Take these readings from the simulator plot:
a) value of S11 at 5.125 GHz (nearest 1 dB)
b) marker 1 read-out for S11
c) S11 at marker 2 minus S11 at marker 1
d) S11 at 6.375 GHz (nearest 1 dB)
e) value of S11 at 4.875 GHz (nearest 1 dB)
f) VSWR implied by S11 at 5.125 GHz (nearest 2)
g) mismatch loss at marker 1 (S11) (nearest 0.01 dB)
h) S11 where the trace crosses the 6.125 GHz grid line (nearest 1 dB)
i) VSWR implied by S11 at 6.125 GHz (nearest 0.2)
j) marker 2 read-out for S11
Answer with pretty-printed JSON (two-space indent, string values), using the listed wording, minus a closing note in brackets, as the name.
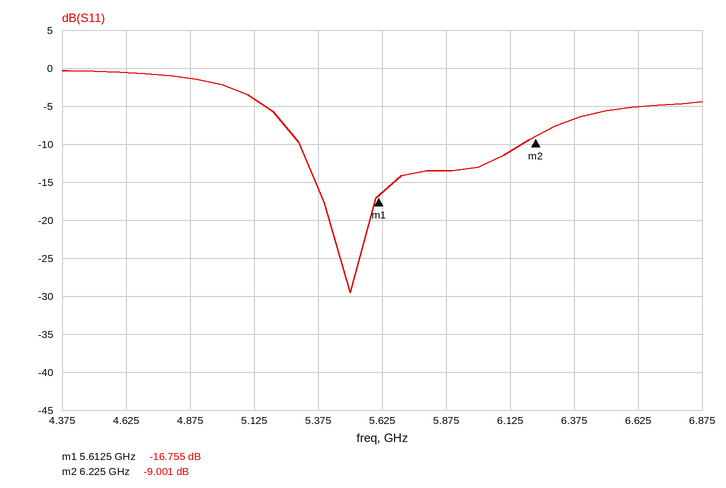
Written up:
{
  "value of S11 at 5.125 GHz": "-4 dB",
  "marker 1 read-out for S11": "-16.755 dB",
  "S11 at marker 2 minus S11 at marker 1": "7.754 dB",
  "S11 at 6.375 GHz": "-7 dB",
  "value of S11 at 4.875 GHz": "-1 dB",
  "VSWR implied by S11 at 5.125 GHz": "4",
  "mismatch loss at marker 1 (S11)": "0.09 dB",
  "S11 where the trace crosses the 6.125 GHz grid line": "-11 dB",
  "VSWR implied by S11 at 6.125 GHz": "1.8",
  "marker 2 read-out for S11": "-9.001 dB"
}
